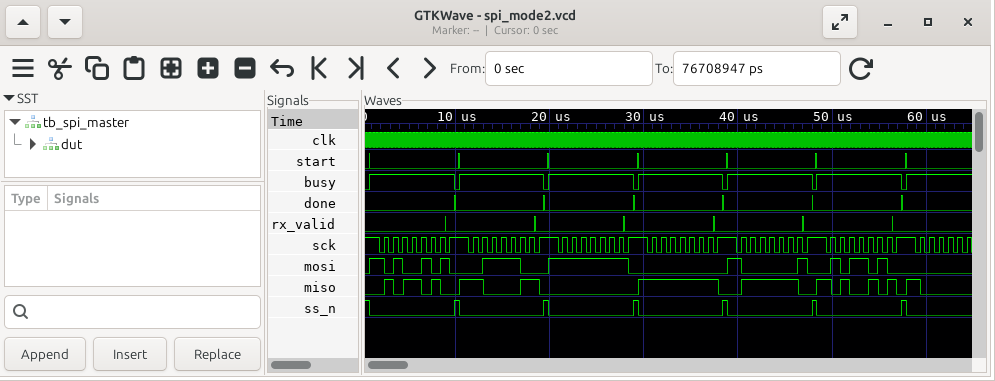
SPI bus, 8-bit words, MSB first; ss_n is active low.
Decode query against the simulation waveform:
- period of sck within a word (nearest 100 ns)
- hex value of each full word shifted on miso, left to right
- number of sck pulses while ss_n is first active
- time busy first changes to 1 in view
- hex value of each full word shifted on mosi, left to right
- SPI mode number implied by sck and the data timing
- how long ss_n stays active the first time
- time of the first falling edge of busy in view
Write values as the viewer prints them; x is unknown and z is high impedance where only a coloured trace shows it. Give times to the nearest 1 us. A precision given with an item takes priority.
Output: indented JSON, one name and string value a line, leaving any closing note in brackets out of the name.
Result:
{
  "period of sck within a word": "1000 ns",
  "hex value of each full word shifted on miso, left to right": "5A, C3, 00, FF, 7E, A5",
  "number of sck pulses while ss_n is first active": "8",
  "time busy first changes to 1 in view": "1 us",
  "hex value of each full word shifted on mosi, left to right": "A5, 3C, FF, 00, 81, 5A",
  "SPI mode number implied by sck and the data timing": "2",
  "how long ss_n stays active the first time": "9 us",
  "time of the first falling edge of busy in view": "10 us"
}
